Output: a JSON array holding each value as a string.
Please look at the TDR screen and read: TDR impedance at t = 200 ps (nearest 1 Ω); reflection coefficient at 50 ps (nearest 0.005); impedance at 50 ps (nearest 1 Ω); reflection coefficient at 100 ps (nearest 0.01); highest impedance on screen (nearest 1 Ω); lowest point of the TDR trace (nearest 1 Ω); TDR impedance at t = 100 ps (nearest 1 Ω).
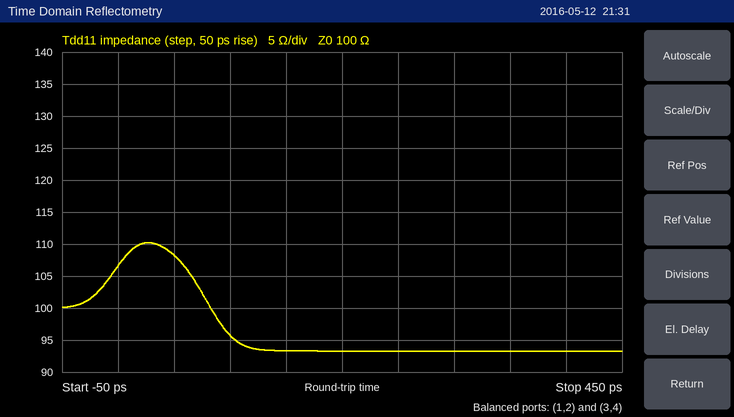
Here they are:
["93 Ω", "+0.040", "108 Ω", "-0.02", "110 Ω", "93 Ω", "96 Ω"]
